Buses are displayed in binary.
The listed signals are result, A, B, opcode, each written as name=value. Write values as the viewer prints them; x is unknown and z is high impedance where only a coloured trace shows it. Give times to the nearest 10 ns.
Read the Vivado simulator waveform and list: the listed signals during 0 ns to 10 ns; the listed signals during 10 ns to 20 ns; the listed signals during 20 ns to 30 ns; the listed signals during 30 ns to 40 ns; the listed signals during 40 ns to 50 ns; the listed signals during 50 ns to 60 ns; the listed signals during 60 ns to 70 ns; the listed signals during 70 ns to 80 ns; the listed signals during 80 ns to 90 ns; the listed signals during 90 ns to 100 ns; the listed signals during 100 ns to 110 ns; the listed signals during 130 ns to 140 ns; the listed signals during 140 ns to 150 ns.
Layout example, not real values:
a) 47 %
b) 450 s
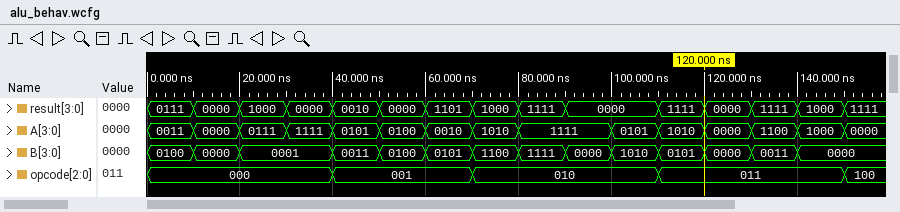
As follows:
a) result=0111, A=0011, B=0100, opcode=000
b) result=0000, A=0000, B=0000, opcode=000
c) result=1000, A=0111, B=0001, opcode=000
d) result=0000, A=1111, B=0001, opcode=000
e) result=0010, A=0101, B=0011, opcode=001
f) result=0000, A=0100, B=0100, opcode=001
g) result=1101, A=0010, B=0101, opcode=001
h) result=1000, A=1010, B=1100, opcode=010
i) result=1111, A=1111, B=1111, opcode=010
j) result=0000, A=1111, B=0000, opcode=010
k) result=0000, A=0101, B=1010, opcode=010
l) result=1111, A=1100, B=0011, opcode=011
m) result=1000, A=1000, B=0000, opcode=011
